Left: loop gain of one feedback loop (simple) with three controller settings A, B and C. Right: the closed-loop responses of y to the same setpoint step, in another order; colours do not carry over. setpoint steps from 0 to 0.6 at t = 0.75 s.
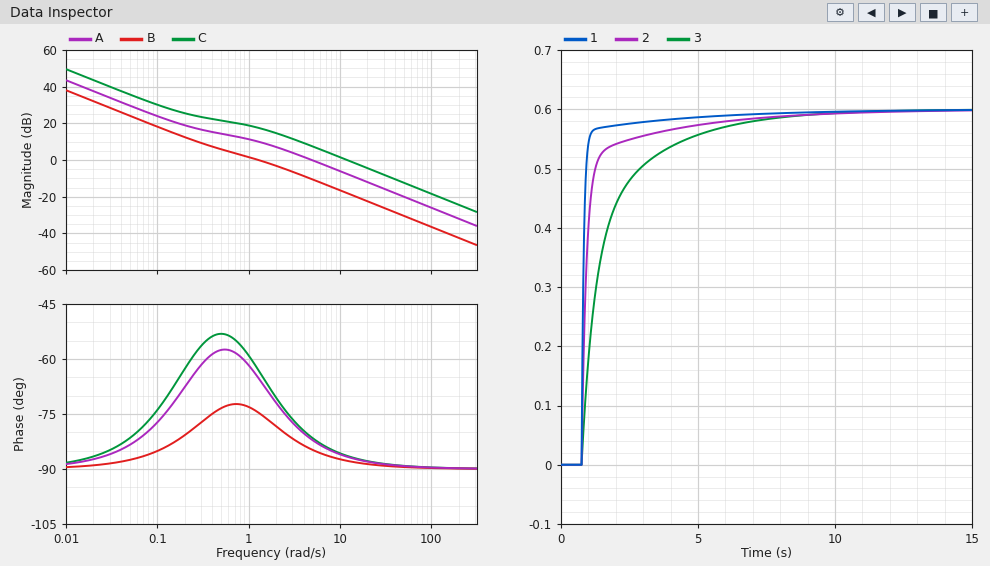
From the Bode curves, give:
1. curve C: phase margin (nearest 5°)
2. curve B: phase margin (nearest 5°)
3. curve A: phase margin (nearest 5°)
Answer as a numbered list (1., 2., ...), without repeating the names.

1. 95°
2. 105°
3. 100°
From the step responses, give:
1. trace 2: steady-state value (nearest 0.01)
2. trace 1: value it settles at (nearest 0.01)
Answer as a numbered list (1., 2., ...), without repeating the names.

1. 0.60
2. 0.60
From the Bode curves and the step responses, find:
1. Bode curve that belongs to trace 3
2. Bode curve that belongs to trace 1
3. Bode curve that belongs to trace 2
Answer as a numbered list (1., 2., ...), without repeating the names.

1. B
2. C
3. A
